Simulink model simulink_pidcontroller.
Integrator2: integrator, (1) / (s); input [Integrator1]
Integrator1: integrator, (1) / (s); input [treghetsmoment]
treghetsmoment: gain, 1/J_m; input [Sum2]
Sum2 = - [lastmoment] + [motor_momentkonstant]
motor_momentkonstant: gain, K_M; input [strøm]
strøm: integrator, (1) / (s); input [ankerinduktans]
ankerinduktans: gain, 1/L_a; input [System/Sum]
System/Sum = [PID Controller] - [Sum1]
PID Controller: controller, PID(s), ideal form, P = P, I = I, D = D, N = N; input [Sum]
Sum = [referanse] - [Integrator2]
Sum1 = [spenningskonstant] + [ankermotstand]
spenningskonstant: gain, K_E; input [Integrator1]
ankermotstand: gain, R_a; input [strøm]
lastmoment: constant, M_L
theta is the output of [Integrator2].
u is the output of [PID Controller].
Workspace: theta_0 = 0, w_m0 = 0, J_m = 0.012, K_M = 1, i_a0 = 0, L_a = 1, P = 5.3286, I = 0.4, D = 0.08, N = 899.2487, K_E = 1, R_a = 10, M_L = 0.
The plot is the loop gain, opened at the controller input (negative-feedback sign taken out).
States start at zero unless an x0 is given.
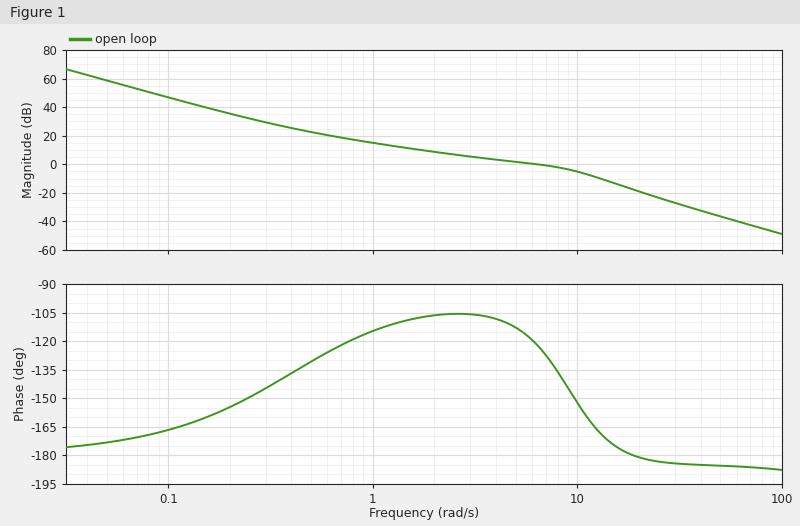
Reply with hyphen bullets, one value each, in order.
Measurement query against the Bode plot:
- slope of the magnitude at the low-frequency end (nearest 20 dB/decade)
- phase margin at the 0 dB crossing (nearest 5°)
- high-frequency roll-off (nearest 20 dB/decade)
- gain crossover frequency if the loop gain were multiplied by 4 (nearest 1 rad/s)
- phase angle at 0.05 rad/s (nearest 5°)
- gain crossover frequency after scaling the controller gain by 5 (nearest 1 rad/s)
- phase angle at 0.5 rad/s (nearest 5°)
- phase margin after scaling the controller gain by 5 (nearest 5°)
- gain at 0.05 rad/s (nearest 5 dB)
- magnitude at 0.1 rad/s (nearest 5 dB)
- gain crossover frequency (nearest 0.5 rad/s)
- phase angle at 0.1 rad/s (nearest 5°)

- -40 dB/decade
- 60°
- -40 dB/decade
- 14 rad/s
- -175°
- 16 rad/s
- -130°
- 5°
- 60 dB
- 45 dB
- 6.5 rad/s
- -165°
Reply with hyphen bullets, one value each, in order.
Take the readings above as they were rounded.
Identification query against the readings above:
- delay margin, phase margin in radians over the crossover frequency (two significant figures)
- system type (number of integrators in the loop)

- 0.16 s
- 2
